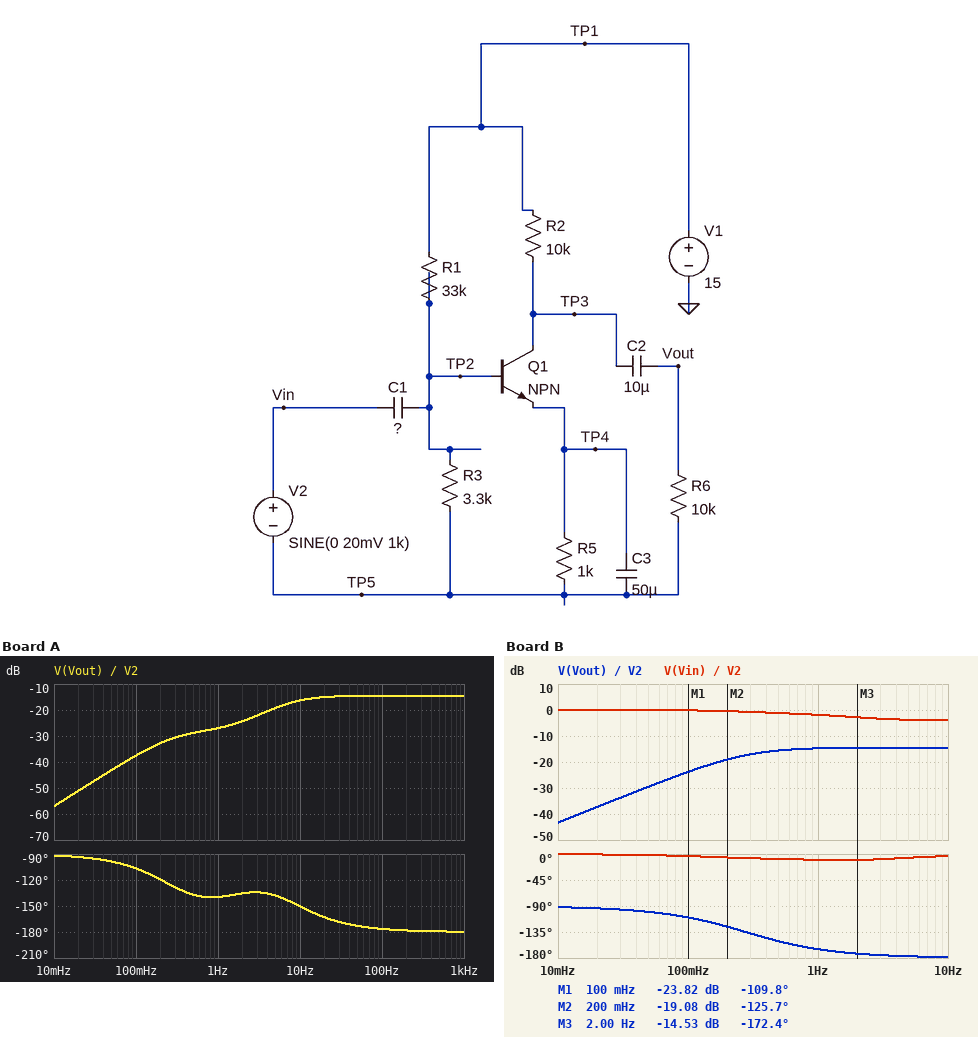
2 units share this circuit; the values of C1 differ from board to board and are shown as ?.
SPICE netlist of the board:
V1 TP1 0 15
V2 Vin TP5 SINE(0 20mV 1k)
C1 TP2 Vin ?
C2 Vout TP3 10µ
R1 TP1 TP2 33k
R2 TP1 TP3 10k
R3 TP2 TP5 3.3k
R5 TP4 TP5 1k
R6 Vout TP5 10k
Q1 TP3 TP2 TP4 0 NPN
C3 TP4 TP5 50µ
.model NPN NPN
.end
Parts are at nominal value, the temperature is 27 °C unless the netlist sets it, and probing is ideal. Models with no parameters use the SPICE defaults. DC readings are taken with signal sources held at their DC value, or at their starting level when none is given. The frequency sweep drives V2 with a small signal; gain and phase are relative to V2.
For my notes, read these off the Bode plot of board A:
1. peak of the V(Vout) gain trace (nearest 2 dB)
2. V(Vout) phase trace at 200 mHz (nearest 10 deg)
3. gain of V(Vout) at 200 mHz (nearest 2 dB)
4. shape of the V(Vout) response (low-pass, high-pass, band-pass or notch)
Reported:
-14 dB
-120 deg
-32 dB
high-pass
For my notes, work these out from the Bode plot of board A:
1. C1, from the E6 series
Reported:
6.8 µF
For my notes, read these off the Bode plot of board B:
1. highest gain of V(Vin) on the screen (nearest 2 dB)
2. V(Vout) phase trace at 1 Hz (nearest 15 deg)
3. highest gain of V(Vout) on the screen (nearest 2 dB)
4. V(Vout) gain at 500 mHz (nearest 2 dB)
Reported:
0 dB
-165 deg
-14 dB
-16 dB
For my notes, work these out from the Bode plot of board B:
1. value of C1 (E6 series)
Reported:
33 µF
